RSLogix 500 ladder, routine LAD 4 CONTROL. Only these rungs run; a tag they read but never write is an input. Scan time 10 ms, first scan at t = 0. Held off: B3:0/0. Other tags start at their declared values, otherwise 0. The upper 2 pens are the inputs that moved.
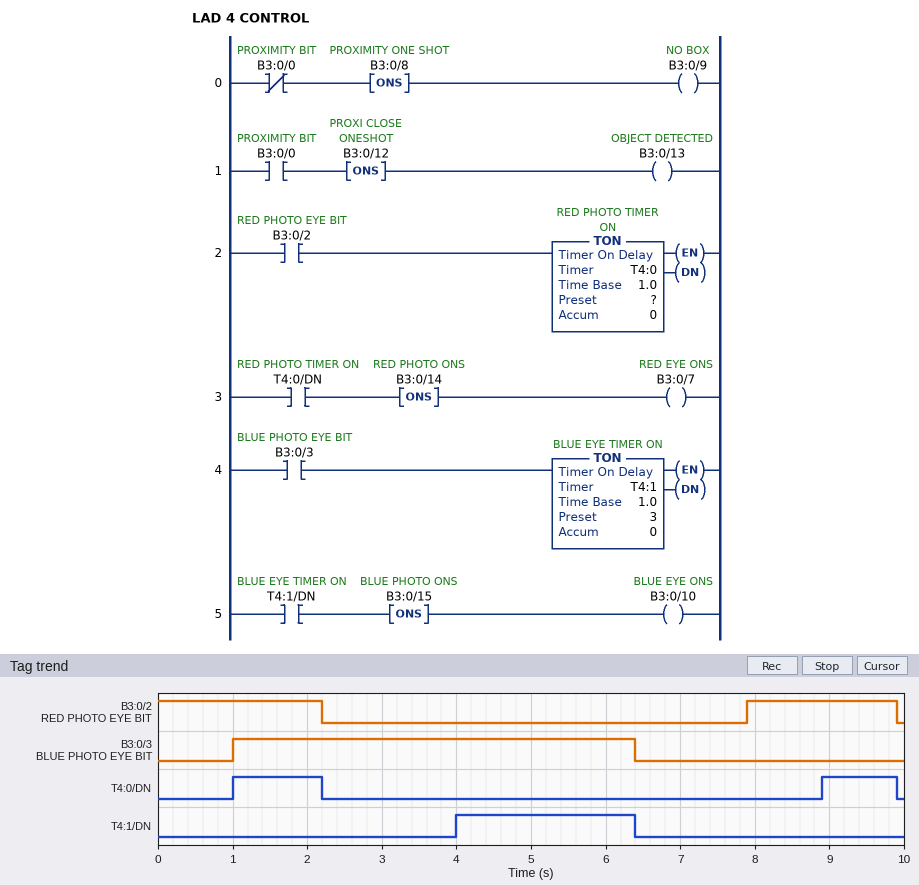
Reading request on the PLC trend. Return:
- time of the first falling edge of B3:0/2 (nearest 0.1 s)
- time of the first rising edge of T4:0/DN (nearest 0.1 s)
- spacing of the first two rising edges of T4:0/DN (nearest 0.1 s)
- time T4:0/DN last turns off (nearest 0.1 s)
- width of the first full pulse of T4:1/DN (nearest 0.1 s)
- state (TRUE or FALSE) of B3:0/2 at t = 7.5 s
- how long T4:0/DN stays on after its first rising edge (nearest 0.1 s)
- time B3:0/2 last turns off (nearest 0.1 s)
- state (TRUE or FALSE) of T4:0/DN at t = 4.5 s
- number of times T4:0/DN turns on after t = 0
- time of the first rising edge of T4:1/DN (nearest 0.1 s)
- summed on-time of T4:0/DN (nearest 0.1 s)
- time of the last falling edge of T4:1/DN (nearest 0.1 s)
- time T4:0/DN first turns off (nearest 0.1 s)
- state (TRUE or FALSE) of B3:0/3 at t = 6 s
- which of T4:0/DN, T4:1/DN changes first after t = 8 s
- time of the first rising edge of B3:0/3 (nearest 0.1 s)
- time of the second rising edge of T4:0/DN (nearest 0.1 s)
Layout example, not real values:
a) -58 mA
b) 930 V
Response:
a) 2.2 s
b) 1.0 s
c) 7.9 s
d) 9.9 s
e) 2.4 s
f) FALSE
g) 1.2 s
h) 9.9 s
i) FALSE
j) 2
k) 4.0 s
l) 2.2 s
m) 6.4 s
n) 2.2 s
o) TRUE
p) T4:0/DN
q) 1.0 s
r) 8.9 s
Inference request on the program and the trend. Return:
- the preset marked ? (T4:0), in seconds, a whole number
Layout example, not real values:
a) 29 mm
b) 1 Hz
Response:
a) 1 s
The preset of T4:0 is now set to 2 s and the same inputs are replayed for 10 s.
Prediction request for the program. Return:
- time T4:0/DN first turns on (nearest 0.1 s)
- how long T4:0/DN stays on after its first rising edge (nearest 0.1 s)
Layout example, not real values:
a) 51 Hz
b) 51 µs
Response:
a) 2.0 s
b) 0.2 s
